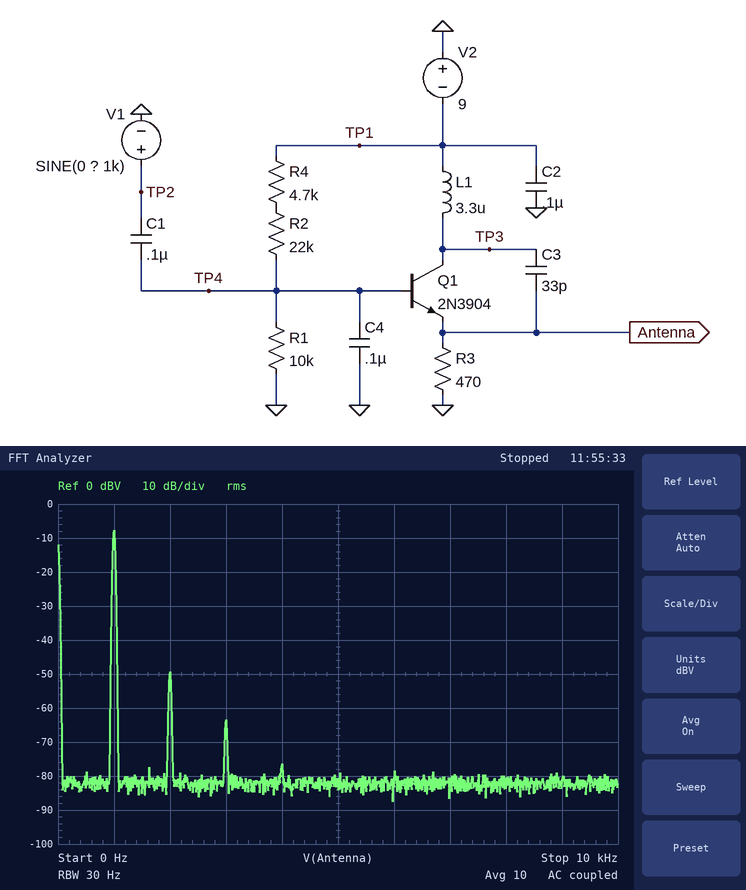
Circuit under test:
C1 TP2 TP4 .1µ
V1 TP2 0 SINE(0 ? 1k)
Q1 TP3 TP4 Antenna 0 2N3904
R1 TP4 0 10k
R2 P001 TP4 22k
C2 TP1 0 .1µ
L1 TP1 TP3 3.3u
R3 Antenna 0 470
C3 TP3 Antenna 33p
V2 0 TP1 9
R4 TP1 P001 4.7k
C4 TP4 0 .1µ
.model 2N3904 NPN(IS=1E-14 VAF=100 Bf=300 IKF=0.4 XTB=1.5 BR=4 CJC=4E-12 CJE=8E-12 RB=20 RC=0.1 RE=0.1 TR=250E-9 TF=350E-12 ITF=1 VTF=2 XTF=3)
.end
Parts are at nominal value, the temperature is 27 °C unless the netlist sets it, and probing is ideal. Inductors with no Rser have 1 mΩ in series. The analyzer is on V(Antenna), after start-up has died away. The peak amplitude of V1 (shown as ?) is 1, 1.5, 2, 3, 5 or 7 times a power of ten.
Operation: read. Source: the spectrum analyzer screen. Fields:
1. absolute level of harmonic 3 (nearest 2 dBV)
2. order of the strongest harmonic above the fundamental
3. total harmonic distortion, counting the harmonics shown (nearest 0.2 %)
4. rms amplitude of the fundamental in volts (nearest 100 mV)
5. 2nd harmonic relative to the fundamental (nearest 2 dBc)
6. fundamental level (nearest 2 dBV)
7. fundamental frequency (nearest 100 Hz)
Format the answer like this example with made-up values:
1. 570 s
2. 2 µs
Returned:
1. -64 dBV
2. 2
3. 0.8 %
4. 400 mV
5. -42 dBc
6. -8 dBV
7. 1.0 kHz
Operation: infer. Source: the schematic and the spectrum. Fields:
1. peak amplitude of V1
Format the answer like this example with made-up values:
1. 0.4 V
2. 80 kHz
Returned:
1. 500 mV
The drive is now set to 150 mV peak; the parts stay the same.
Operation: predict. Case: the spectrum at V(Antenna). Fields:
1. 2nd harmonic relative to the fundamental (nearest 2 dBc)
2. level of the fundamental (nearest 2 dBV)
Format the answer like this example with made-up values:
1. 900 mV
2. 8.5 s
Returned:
1. -52 dBc
2. -18 dBV
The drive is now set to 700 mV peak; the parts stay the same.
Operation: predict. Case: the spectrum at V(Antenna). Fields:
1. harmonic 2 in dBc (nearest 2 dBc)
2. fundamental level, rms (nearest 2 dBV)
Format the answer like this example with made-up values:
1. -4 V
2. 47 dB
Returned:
1. -38 dBc
2. -4 dBV
